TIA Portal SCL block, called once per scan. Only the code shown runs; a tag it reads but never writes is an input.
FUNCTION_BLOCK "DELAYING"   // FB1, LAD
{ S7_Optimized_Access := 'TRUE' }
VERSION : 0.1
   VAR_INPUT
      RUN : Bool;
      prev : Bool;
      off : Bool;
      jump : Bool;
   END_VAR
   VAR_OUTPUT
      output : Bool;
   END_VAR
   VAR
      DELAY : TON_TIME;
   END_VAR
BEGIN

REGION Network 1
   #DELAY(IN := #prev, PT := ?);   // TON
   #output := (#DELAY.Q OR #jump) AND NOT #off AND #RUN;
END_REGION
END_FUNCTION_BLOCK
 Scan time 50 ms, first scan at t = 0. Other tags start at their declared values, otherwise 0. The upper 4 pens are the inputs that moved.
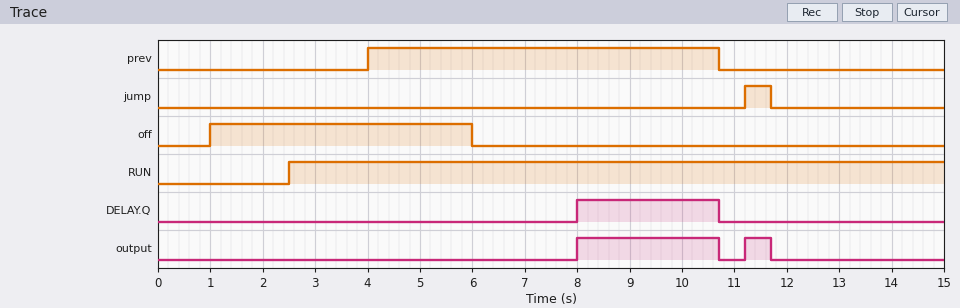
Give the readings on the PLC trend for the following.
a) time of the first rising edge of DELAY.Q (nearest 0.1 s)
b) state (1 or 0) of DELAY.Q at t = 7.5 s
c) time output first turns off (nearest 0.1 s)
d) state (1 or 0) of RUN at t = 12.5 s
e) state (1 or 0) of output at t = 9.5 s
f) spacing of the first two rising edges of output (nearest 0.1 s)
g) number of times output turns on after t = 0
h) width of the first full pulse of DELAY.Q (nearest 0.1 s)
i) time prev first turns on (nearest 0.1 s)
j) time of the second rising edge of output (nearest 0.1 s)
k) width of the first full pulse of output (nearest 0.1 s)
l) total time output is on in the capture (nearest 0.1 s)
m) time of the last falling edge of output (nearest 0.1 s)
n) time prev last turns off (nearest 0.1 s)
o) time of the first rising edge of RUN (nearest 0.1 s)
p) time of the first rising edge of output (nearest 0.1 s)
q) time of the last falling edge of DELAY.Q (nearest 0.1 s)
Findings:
8.0 s
0
10.7 s
1
1
3.2 s
2
2.7 s
4.0 s
11.2 s
2.7 s
3.2 s
11.7 s
10.7 s
2.5 s
8.0 s
10.7 s
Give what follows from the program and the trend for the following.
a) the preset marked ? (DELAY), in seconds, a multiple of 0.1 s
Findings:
4.0 s
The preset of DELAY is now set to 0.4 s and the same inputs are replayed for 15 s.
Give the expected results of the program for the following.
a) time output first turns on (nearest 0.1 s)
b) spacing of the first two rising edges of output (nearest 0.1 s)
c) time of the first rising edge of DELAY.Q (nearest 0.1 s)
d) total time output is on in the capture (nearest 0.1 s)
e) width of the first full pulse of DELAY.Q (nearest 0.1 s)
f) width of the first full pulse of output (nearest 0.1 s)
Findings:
6.0 s
5.2 s
4.4 s
5.2 s
6.3 s
4.7 s
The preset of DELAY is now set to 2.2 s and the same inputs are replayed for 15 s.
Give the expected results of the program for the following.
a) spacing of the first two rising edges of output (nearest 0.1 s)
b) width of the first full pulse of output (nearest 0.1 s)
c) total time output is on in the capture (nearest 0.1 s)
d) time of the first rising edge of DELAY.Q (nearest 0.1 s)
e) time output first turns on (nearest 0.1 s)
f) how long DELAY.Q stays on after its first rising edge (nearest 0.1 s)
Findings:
5.0 s
4.5 s
5.0 s
6.2 s
6.2 s
4.5 s
